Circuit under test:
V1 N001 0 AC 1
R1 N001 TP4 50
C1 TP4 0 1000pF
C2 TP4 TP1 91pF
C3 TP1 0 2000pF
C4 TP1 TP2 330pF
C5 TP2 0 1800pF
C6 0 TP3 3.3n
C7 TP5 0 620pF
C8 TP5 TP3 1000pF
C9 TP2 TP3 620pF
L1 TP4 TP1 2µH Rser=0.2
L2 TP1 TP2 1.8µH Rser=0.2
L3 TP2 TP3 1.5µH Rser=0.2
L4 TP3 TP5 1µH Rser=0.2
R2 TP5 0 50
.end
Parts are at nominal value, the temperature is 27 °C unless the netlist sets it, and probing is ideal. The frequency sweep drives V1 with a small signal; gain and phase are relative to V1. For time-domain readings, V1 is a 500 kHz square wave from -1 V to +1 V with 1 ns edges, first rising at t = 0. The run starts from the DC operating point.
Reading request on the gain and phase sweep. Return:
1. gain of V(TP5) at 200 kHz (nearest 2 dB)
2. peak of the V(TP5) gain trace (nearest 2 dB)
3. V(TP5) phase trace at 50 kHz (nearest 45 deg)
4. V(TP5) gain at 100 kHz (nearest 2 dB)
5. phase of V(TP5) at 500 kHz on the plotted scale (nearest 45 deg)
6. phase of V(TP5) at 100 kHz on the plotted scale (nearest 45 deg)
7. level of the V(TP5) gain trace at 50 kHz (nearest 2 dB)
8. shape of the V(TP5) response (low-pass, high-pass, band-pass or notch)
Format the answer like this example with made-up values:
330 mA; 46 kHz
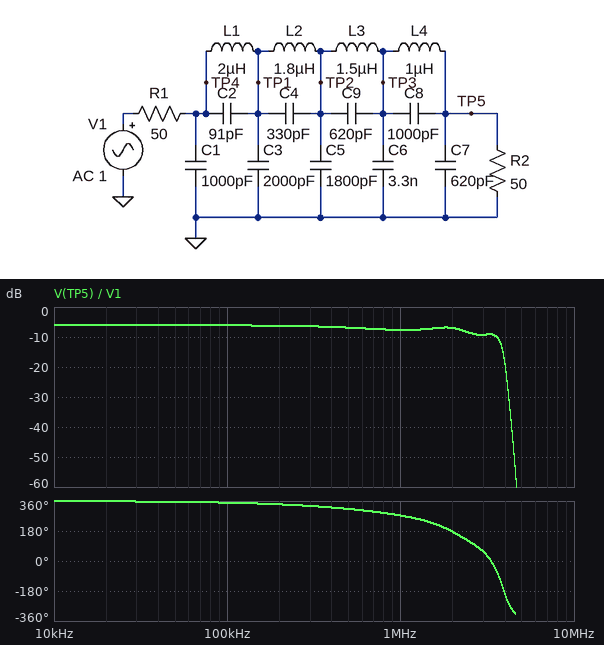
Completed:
-6 dB; -6 dB; 360 deg; -6 dB; 315 deg; 360 deg; -6 dB; low-pass
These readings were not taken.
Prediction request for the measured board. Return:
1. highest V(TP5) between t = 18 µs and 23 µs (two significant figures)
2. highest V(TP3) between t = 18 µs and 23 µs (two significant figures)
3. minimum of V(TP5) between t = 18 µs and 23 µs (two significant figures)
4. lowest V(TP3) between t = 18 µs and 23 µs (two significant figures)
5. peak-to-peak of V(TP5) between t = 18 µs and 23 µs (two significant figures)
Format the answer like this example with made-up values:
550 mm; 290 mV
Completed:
570 mV; 530 mV; -570 mV; -530 mV; 1.1 V
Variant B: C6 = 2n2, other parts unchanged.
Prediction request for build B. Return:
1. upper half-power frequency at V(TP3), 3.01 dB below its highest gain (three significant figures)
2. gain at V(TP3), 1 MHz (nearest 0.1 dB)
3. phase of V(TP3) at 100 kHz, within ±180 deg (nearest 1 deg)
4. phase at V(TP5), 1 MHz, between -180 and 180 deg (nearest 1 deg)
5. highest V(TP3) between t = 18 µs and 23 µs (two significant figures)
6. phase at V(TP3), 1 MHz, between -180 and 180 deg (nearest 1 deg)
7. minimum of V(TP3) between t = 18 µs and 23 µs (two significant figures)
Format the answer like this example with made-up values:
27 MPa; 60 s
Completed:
3.95 MHz; -7.4 dB; -8 deg; -82 deg; 570 mV; -74 deg; -570 mV
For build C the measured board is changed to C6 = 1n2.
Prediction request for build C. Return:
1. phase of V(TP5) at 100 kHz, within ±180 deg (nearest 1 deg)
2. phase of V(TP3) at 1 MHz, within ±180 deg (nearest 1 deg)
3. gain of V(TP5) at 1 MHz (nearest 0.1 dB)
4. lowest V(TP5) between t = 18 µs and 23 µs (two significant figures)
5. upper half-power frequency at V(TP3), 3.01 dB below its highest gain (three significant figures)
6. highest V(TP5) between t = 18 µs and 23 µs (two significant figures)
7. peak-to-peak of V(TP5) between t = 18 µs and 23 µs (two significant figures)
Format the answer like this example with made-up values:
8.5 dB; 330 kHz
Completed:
-8 deg; -69 deg; -6.9 dB; -640 mV; 4.19 MHz; 640 mV; 1.3 V
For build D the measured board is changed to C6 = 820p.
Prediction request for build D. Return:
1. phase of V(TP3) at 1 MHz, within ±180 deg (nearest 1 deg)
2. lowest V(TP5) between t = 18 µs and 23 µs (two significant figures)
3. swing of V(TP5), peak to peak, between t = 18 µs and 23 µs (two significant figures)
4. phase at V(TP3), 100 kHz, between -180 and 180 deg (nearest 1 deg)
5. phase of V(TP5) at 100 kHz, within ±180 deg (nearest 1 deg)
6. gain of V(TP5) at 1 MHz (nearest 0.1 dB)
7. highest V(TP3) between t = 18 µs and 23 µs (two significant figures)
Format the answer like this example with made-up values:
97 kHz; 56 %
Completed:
-67 deg; -640 mV; 1.3 V; -7 deg; -8 deg; -6.8 dB; 580 mV
